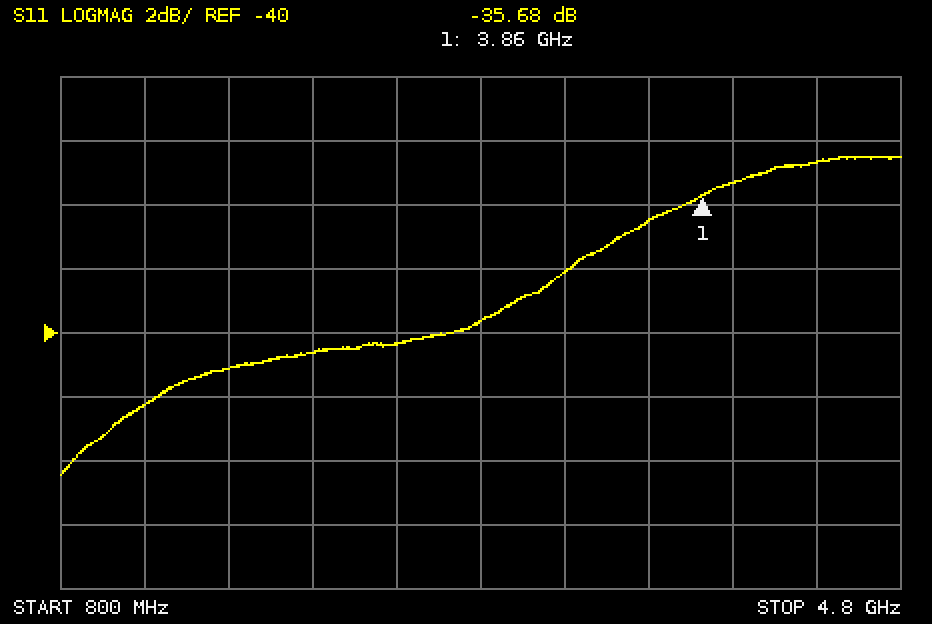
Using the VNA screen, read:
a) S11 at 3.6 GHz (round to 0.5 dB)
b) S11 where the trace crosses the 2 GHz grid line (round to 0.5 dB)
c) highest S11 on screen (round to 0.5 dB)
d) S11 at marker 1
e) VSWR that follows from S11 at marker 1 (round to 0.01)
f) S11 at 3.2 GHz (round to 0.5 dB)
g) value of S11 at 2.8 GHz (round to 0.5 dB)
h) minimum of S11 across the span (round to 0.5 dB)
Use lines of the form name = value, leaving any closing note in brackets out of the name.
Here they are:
S11 at 3.6 GHz = -36.5 dB
S11 where the trace crosses the 2 GHz grid line = -40.5 dB
highest S11 on screen = -34.5 dB
S11 at marker 1 = -35.68 dB
VSWR that follows from S11 at marker 1 = 1.03
S11 at 3.2 GHz = -38.0 dB
value of S11 at 2.8 GHz = -39.5 dB
minimum of S11 across the span = -44.5 dB
